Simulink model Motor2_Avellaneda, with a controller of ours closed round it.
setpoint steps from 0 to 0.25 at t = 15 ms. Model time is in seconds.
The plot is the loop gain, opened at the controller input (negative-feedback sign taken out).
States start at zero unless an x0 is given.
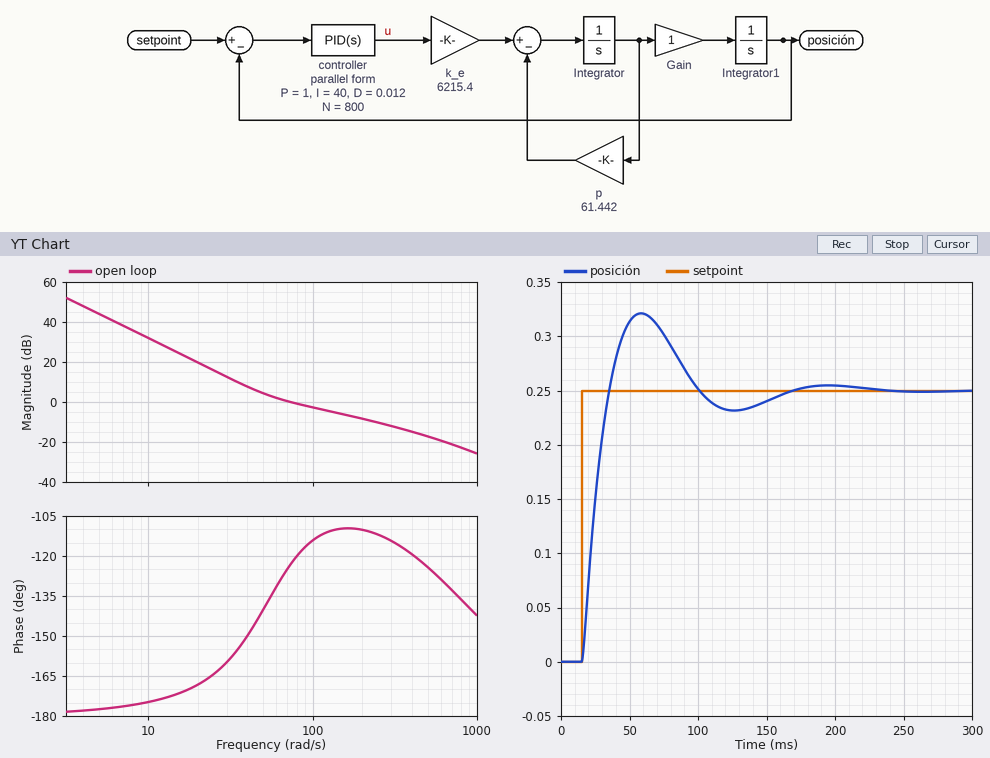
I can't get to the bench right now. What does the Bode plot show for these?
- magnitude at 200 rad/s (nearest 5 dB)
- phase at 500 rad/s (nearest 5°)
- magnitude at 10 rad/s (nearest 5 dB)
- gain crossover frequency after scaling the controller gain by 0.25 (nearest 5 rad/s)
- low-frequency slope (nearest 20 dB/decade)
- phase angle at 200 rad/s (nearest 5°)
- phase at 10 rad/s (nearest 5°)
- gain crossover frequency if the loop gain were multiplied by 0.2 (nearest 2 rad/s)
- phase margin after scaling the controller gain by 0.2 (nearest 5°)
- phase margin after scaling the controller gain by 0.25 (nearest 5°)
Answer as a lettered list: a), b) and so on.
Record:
a) -10 dB
b) -125°
c) 30 dB
d) 30 rad/s
e) -40 dB/decade
f) -110°
g) -175°
h) 28 rad/s
i) 20°
j) 20°
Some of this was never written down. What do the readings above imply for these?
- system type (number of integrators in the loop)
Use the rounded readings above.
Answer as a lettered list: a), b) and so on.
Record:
a) 2
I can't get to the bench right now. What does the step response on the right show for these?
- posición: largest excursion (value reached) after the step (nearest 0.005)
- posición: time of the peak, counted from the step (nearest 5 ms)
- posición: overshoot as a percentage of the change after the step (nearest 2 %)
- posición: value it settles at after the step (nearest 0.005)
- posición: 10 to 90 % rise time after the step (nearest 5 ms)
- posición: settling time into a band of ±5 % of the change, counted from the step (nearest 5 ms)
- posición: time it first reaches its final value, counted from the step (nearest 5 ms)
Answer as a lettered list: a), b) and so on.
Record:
a) 0.320
b) 45 ms
c) 28 %
d) 0.250
e) 15 ms
f) 130 ms
g) 20 ms
